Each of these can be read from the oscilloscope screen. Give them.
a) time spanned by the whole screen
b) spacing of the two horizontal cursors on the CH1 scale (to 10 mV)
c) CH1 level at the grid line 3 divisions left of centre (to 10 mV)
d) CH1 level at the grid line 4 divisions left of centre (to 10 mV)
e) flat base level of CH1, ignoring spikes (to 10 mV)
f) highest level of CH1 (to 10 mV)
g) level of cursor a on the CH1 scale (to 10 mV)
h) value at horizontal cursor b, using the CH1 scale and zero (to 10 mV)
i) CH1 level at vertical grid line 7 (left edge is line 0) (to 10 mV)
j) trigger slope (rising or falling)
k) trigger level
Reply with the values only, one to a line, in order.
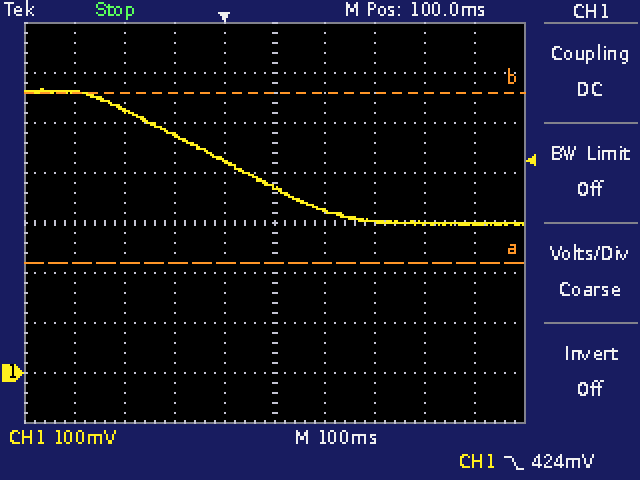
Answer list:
1 s
340 mV
530 mV
560 mV
300 mV
570 mV
220 mV
560 mV
300 mV
falling
424 mV
